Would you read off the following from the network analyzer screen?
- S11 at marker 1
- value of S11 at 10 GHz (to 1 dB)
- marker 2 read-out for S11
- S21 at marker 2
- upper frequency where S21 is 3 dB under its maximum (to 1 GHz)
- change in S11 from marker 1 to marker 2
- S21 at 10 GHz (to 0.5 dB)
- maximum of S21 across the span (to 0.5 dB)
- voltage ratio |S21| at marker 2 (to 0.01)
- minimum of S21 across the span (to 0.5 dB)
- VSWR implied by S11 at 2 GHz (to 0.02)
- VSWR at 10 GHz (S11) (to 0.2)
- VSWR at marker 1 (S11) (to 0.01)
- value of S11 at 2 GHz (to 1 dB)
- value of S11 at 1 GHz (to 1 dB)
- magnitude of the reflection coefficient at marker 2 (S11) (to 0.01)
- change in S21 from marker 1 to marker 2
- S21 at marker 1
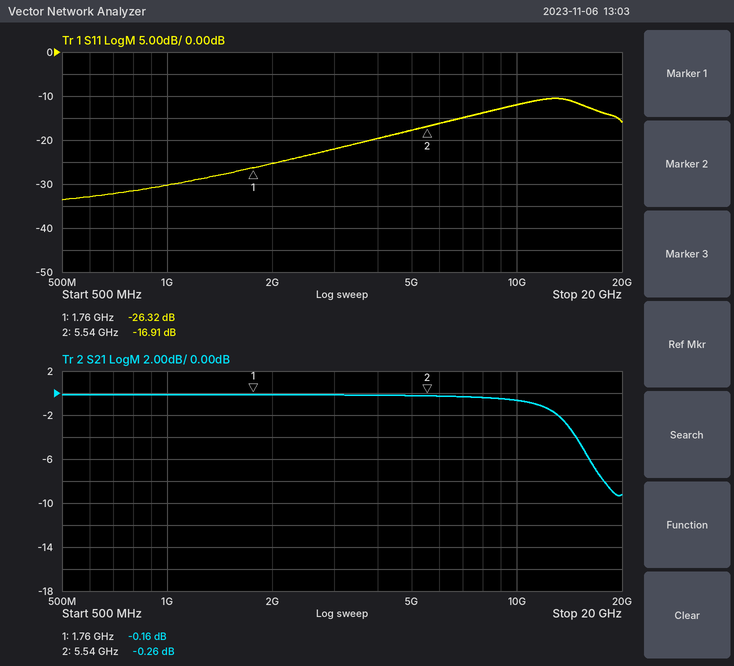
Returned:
-26.32 dB
-12 dB
-16.91 dB
-0.26 dB
14 GHz
9.41 dB
-0.5 dB
0.0 dB
0.97
-9.5 dB
1.12
1.6
1.10
-25 dB
-30 dB
0.14
-0.10 dB
-0.16 dB
